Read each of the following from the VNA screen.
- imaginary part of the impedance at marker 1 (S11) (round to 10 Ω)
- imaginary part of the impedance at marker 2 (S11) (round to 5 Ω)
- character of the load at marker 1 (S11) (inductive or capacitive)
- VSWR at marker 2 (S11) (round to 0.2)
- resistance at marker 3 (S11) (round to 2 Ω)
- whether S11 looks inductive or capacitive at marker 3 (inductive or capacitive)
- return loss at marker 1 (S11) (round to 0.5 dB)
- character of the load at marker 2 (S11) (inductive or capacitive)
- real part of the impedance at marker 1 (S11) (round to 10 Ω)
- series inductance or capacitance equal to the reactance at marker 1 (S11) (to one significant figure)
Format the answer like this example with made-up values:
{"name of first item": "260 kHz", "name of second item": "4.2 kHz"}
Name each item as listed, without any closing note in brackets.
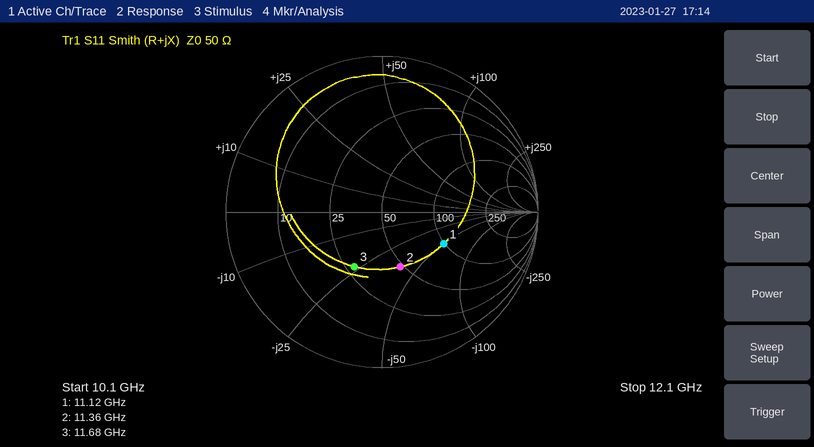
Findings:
{"imaginary part of the impedance at marker 1 (S11)": "-50 Ω", "imaginary part of the impedance at marker 2 (S11)": "-40 Ω", "character of the load at marker 1 (S11)": "capacitive", "VSWR at marker 2 (S11)": "2.2", "resistance at marker 3 (S11)": "28 Ω", "whether S11 looks inductive or capacitive at marker 3": "capacitive", "return loss at marker 1 (S11)": "7.0 dB", "character of the load at marker 2 (S11)": "capacitive", "real part of the impedance at marker 1 (S11)": "100 Ω", "series inductance or capacitance equal to the reactance at marker 1 (S11)": "300 fF"}
